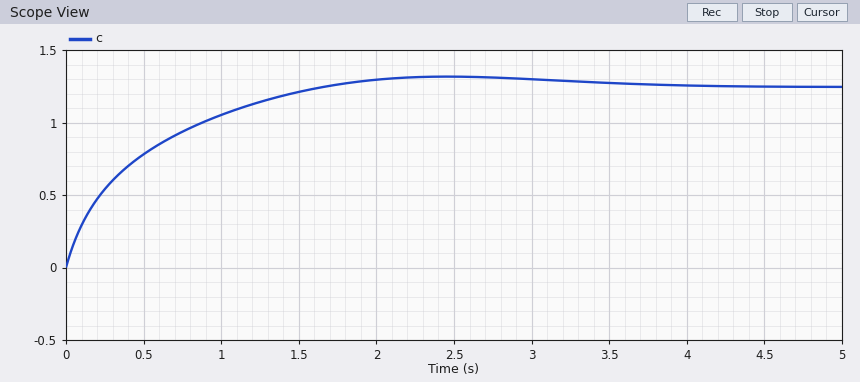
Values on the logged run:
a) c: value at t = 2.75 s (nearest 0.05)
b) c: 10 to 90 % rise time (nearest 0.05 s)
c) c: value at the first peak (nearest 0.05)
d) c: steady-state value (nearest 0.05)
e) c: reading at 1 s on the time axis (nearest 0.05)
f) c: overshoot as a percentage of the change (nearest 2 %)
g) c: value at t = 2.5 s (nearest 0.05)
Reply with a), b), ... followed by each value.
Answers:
a) 1.30
b) 1.15 s
c) 1.30
d) 1.25
e) 1.05
f) 6 %
g) 1.30
